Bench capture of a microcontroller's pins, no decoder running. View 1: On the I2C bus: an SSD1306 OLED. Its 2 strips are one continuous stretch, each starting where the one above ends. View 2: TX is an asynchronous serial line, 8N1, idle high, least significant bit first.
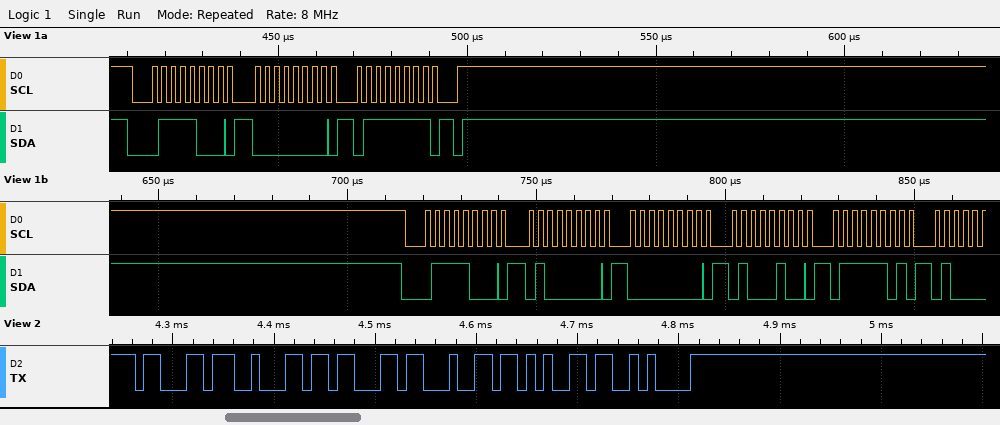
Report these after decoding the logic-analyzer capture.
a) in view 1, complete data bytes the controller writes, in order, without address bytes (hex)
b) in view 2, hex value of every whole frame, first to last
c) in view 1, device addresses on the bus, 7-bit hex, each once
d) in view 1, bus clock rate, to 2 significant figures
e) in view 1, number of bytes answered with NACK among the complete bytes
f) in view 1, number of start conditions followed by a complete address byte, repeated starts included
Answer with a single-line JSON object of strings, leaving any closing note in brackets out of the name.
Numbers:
{"in view 1, complete data bytes the controller writes, in order, without address bytes": "00 7F 40 00 44 7D", "in view 2, hex value of every whole frame, first to last": "63 62 63 64 65 0A", "in view 1, device addresses on the bus, 7-bit hex, each once": "0x3C", "in view 1, bus clock rate, to 2 significant figures": "400 kHz", "in view 1, number of bytes answered with NACK among the complete bytes": "0", "in view 1, number of start conditions followed by a complete address byte, repeated starts included": "2"}
